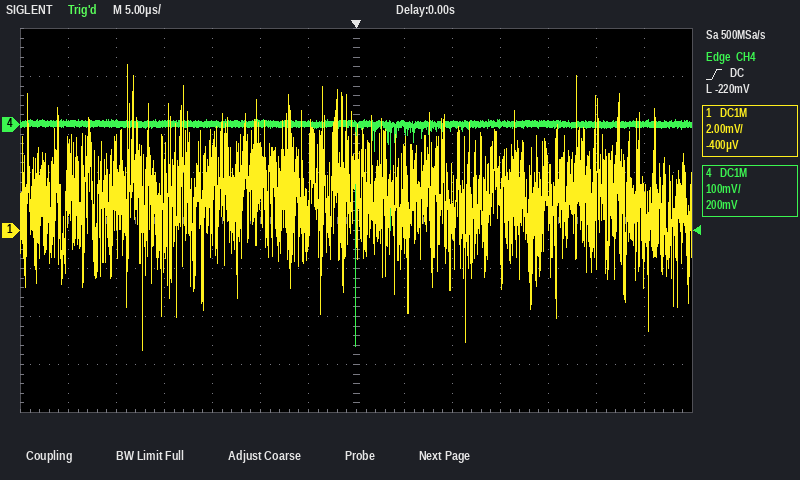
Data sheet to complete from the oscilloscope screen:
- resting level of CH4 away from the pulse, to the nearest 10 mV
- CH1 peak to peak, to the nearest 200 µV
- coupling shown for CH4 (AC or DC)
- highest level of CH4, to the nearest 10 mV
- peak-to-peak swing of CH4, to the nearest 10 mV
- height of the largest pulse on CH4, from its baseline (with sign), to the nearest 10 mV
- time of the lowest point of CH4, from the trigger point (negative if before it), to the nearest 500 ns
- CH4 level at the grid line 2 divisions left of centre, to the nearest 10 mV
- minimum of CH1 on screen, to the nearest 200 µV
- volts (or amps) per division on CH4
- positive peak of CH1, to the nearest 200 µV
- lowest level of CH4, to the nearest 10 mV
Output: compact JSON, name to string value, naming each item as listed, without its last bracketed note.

{"resting level of CH4 away from the pulse, to the nearest 10 mV": "0 mV", "CH1 peak to peak, to the nearest 200 µV": "11.8 mV", "coupling shown for CH4": "DC", "highest level of CH4, to the nearest 10 mV": "10 mV", "peak-to-peak swing of CH4, to the nearest 10 mV": "470 mV", "height of the largest pulse on CH4, from its baseline (with sign), to the nearest 10 mV": "-460 mV", "time of the lowest point of CH4, from the trigger point (negative if before it), to the nearest 500 ns": "0.0 µs", "CH4 level at the grid line 2 divisions left of centre, to the nearest 10 mV": "0 mV", "minimum of CH1 on screen, to the nearest 200 µV": "-5.0 mV", "volts (or amps) per division on CH4": "100 mV", "positive peak of CH1, to the nearest 200 µV": "6.8 mV", "lowest level of CH4, to the nearest 10 mV": "-460 mV"}
